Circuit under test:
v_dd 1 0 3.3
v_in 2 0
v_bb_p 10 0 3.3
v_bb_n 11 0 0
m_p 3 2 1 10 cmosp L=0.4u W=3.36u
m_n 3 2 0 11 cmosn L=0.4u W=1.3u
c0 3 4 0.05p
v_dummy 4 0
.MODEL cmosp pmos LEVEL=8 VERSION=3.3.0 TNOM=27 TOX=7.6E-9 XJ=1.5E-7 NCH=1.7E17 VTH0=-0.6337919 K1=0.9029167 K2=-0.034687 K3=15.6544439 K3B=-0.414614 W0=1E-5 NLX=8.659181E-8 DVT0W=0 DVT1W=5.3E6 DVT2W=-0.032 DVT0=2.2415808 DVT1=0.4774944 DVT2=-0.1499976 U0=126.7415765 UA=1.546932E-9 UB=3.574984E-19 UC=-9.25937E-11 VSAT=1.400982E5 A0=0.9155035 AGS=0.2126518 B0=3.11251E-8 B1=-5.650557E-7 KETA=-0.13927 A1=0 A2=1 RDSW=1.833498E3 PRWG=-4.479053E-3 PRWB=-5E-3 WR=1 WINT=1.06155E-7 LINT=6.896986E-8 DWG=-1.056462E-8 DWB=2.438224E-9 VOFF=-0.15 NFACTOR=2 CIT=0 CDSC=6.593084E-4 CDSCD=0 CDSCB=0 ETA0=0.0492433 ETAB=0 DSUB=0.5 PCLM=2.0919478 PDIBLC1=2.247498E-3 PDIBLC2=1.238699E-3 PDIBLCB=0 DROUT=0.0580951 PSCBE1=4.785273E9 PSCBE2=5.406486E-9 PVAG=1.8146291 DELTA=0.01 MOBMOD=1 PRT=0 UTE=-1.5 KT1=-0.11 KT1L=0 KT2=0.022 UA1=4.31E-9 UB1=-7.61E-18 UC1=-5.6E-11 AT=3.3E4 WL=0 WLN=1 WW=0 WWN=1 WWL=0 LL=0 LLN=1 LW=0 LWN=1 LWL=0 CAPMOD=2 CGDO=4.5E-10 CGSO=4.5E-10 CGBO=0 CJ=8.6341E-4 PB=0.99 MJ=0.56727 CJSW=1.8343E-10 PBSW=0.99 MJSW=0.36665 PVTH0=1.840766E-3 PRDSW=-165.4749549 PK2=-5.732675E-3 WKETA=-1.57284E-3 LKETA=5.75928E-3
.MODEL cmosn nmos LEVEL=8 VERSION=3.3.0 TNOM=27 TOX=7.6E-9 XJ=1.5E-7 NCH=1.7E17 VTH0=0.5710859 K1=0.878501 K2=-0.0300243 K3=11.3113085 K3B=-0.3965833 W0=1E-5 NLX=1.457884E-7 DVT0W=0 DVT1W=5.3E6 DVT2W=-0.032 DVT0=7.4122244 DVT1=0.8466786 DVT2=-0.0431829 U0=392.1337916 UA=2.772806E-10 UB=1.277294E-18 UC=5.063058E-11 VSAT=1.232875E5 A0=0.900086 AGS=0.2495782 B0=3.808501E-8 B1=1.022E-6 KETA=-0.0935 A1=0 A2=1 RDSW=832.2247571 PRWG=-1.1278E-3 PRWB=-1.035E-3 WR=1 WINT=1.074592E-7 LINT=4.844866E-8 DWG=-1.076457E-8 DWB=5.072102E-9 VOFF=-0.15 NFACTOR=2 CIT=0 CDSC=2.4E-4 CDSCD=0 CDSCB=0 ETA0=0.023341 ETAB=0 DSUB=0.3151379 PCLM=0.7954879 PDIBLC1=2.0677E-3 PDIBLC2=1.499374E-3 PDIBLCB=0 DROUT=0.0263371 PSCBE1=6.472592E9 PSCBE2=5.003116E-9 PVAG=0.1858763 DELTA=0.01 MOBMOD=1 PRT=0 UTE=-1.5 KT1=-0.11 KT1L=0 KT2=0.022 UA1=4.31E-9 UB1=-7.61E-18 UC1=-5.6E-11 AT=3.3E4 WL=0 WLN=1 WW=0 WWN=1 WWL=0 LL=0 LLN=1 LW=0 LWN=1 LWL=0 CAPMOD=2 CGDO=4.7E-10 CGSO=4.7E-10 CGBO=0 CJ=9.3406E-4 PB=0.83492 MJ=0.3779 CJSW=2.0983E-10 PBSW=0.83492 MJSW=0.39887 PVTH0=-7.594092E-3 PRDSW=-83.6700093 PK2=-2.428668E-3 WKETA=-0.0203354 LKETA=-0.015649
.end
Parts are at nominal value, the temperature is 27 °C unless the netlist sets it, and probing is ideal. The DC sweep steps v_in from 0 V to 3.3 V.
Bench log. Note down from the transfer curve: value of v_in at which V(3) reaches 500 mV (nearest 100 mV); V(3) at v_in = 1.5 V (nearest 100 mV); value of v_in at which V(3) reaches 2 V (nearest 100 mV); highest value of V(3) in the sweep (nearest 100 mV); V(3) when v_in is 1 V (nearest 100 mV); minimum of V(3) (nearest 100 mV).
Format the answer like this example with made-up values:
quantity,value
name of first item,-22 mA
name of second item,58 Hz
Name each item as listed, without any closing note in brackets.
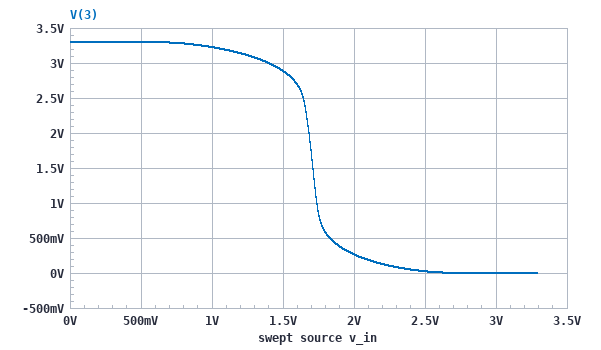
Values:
quantity,value
value of v_in at which V(3) reaches 500 mV,1.8 V
V(3) at v_in = 1.5 V,2.9 V
value of v_in at which V(3) reaches 2 V,1.7 V
highest value of V(3) in the sweep,3.3 V
V(3) when v_in is 1 V,3.2 V
minimum of V(3),0 V
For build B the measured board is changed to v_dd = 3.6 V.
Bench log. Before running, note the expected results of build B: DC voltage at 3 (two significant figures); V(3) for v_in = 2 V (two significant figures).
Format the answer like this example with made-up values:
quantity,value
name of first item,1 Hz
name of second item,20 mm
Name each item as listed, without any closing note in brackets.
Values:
quantity,value
DC voltage at 3,3.6 V
V(3) for v_in = 2 V,700 mV
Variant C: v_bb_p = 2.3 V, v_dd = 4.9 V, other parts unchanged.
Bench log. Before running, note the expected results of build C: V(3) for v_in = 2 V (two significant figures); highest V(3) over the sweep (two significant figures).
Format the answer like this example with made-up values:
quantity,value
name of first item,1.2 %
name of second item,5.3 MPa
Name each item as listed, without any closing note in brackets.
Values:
quantity,value
V(3) for v_in = 2 V,2.9 V
highest V(3) over the sweep,3.0 V
